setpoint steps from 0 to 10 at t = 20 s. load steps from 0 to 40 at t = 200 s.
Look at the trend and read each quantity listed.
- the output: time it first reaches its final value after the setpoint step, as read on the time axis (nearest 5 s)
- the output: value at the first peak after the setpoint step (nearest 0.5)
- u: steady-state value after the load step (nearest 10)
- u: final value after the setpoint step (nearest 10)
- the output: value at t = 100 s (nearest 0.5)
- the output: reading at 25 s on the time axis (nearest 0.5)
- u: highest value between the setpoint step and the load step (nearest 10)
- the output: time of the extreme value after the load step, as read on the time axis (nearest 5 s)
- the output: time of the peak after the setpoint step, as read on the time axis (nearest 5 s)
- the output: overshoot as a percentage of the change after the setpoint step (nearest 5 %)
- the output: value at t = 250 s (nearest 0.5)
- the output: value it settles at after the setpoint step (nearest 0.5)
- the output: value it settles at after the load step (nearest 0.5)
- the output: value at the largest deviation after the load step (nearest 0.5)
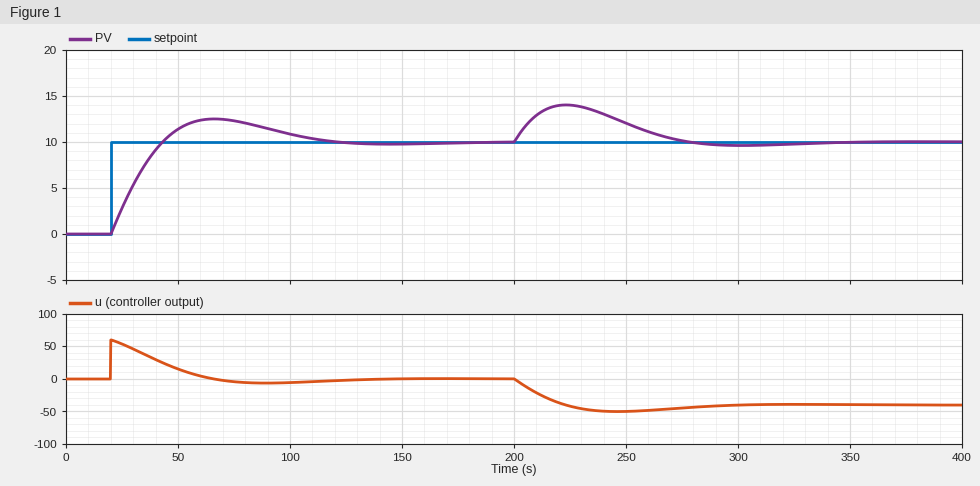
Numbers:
45 s
12.5
-40
0
11.0
3.0
60
225 s
65 s
25 %
12.0
10.0
10.0
14.0
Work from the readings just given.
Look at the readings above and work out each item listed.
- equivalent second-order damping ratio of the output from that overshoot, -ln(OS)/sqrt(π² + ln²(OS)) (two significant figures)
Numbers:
0.40
